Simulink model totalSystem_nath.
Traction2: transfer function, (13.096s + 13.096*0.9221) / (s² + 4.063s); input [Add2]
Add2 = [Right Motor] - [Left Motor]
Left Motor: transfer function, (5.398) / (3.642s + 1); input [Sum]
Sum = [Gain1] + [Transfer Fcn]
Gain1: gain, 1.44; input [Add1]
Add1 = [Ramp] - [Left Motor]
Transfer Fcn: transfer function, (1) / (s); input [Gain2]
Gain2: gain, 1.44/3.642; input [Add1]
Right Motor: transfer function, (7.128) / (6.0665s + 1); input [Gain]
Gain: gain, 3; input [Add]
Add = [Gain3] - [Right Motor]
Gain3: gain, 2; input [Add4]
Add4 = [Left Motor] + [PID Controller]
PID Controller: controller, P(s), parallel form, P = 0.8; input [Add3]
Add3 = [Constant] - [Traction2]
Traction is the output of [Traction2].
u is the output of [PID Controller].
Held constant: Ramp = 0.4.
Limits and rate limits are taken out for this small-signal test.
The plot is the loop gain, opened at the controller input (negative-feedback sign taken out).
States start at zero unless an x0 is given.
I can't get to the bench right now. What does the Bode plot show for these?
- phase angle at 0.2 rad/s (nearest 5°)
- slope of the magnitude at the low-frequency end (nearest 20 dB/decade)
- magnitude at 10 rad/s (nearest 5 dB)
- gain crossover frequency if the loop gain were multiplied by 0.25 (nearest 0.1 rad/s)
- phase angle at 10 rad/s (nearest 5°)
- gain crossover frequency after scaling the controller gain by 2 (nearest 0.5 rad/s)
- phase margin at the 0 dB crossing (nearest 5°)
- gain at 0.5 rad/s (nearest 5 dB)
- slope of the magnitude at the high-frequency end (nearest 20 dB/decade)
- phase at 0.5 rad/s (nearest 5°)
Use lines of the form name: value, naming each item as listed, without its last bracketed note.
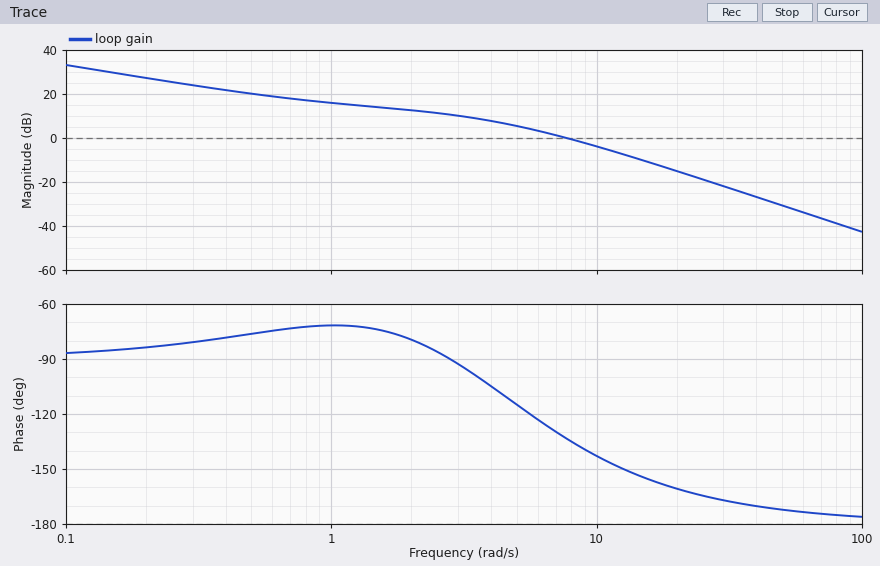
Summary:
phase angle at 0.2 rad/s: -85°
slope of the magnitude at the low-frequency end: -20 dB/decade
magnitude at 10 rad/s: -5 dB
gain crossover frequency if the loop gain were multiplied by 0.25: 2.2 rad/s
phase angle at 10 rad/s: -145°
gain crossover frequency after scaling the controller gain by 2: 11.5 rad/s
phase margin at the 0 dB crossing: 45°
gain at 0.5 rad/s: 20 dB
slope of the magnitude at the high-frequency end: -40 dB/decade
phase at 0.5 rad/s: -75°
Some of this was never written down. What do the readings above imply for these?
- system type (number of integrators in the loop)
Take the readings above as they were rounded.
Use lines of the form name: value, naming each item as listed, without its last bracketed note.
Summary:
system type: 1
